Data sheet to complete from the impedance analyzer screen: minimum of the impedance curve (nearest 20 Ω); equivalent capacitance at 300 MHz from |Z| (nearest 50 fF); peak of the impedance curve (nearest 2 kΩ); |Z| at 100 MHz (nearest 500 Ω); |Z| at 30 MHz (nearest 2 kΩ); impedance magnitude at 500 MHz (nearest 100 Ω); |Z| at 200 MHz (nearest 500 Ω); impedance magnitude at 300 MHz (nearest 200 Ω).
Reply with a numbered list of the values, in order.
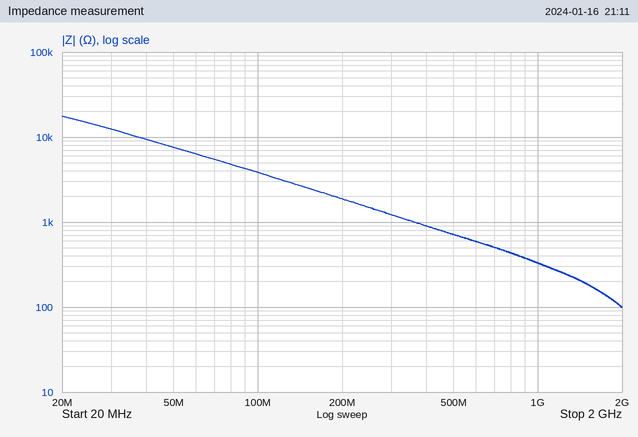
1. 100 Ω
2. 450 fF
3. 18 kΩ
4. 4.0 kΩ
5. 12 kΩ
6. 700 Ω
7. 2.0 kΩ
8. 1.2 kΩ
